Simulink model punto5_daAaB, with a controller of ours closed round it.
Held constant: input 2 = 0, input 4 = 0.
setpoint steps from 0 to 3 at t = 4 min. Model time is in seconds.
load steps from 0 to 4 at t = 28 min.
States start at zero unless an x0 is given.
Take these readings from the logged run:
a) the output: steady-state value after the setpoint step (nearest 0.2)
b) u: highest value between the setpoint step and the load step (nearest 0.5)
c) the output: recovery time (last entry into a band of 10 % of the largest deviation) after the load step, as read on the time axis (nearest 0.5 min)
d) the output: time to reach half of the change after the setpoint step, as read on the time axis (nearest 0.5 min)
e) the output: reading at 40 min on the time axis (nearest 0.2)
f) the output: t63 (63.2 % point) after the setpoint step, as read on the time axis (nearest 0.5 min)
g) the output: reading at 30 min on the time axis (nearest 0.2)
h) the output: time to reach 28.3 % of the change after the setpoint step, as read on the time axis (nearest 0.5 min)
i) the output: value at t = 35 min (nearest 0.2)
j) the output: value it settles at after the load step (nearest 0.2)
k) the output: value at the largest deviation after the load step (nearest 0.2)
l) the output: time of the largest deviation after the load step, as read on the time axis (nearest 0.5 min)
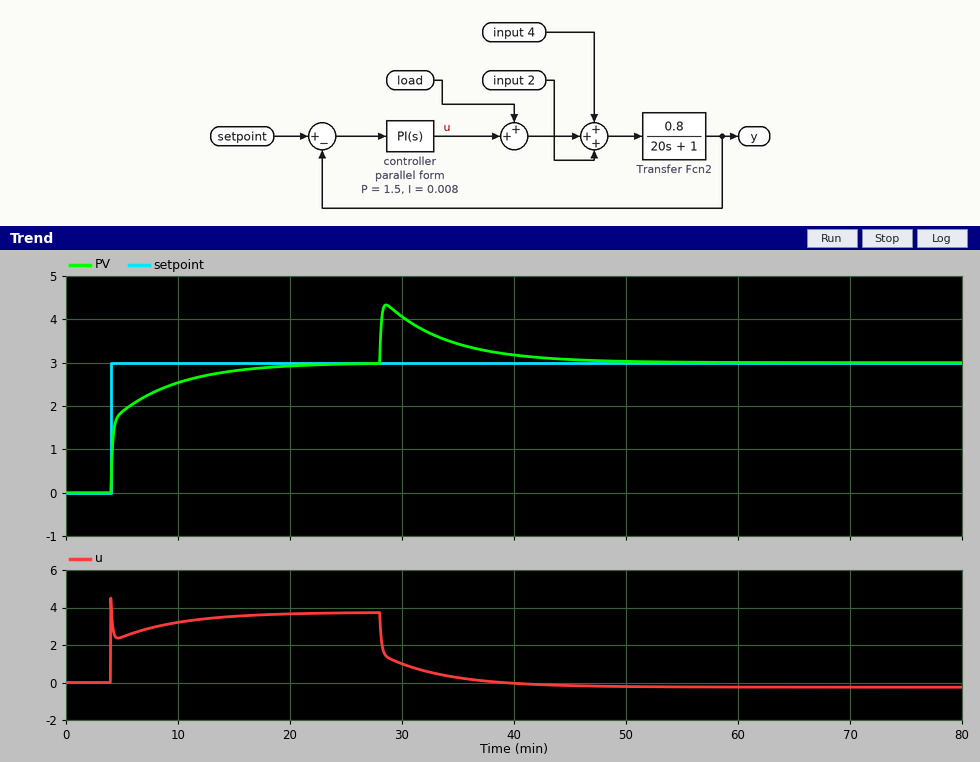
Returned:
3.0
4.5
41.5 min
4.5 min
3.2
5.0 min
4.0
4.0 min
3.4
3.0
4.4
28.5 min
